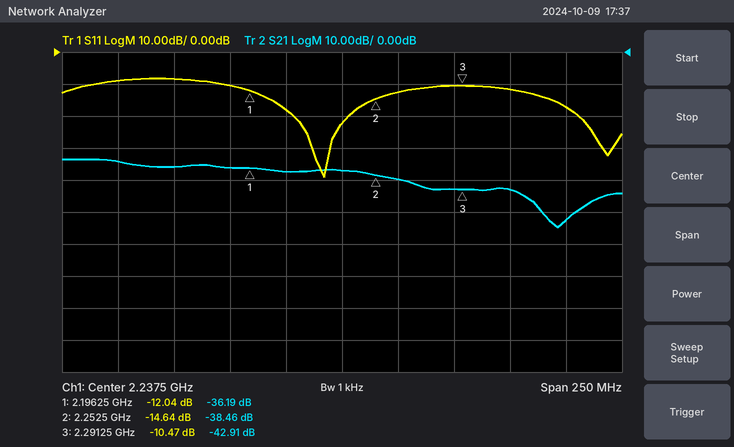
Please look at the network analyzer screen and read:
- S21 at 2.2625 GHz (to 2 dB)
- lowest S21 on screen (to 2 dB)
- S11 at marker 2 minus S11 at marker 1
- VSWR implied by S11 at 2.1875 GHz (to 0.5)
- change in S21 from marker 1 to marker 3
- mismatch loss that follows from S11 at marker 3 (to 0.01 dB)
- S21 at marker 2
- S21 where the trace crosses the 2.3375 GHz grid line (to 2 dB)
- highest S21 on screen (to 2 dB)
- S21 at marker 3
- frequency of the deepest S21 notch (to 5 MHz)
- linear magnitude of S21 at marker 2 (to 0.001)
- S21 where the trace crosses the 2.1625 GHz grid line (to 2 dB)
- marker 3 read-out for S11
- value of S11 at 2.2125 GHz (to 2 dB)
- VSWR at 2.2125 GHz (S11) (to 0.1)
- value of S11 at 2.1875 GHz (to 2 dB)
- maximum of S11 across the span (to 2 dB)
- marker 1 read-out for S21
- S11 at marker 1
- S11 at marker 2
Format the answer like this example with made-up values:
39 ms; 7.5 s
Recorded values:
-40 dB; -54 dB; -2.60 dB; 2.0; -6.72 dB; 0.41 dB; -38.46 dB; -52 dB; -34 dB; -42.91 dB; 2.335 GHz; 0.012; -36 dB; -10.47 dB; -18 dB; 1.3; -10 dB; -8 dB; -36.19 dB; -12.04 dB; -14.64 dB
